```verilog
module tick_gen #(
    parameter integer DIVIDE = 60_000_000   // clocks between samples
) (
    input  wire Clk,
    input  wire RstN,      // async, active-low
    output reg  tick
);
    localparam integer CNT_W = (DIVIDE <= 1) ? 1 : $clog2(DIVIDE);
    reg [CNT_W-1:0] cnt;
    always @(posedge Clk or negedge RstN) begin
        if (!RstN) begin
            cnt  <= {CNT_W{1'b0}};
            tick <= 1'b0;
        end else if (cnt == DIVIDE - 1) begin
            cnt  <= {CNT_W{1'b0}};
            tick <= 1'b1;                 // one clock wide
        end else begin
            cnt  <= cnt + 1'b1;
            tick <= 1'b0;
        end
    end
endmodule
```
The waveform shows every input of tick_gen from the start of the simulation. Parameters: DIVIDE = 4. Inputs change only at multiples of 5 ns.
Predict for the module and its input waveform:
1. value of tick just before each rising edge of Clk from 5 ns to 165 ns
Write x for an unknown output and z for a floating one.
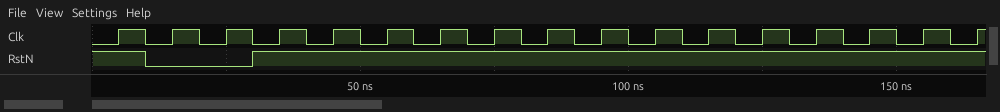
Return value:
x 0 0 0 0 0 0 1 0 0 0 1 0 0 0 1 0
